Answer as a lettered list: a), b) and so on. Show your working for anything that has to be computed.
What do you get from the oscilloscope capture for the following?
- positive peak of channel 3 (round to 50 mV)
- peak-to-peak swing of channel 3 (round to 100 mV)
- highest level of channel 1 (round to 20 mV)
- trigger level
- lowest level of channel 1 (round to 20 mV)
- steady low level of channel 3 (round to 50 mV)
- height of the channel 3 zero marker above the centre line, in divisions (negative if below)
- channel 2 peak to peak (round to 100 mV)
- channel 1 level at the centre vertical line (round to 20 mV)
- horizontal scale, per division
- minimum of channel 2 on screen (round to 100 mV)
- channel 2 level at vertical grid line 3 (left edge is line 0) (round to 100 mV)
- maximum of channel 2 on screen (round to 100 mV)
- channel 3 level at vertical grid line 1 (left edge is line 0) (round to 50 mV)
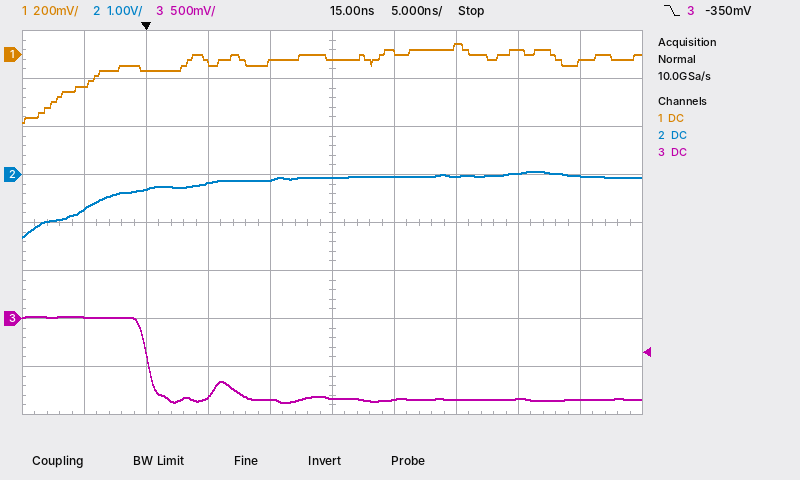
a) 0 mV
b) 900 mV
c) 40 mV
d) -350 mV
e) -280 mV
f) -850 mV
g) -2.0 div
h) 100 mV − (-1.3 V) = 1.4 V
i) -20 mV
j) 5 ns
k) -1.3 V
l) -200 mV
m) 100 mV
n) 0 mV
